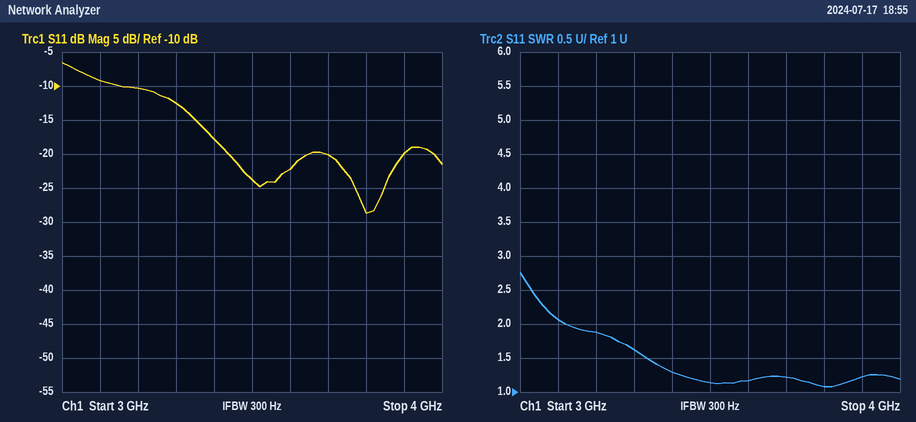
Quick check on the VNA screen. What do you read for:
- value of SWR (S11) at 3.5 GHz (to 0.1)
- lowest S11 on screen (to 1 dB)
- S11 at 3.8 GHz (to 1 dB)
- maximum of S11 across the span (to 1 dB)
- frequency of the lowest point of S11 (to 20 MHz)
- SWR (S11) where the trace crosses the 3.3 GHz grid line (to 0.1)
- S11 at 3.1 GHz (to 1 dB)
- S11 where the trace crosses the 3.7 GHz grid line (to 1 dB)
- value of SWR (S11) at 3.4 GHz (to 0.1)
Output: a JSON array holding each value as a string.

["1.1", "-29 dB", "-29 dB", "-7 dB", "3.80 GHz", "1.6", "-9 dB", "-20 dB", "1.3"]
